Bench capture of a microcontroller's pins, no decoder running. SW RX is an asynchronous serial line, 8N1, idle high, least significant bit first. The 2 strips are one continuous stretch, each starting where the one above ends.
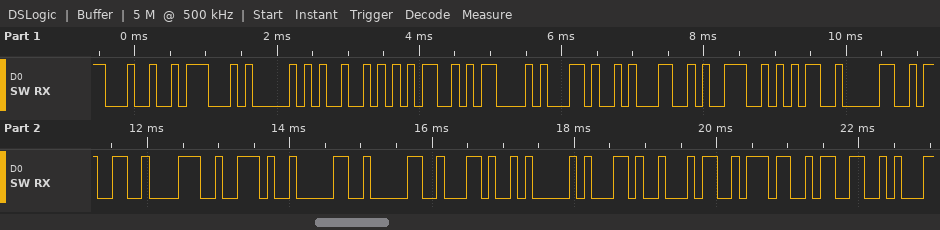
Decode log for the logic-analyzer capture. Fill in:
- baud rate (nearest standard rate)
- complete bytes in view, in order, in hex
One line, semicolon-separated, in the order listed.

9600 baud; 0x24 0x47 0x50 0x52 0x4D 0x43 0x2C 0x31 0x39 0x35 0x30 0x33 0x38 0x2E 0x30 0x30 0x2C 0x41 0x2C 0x34 0x37 0x33
